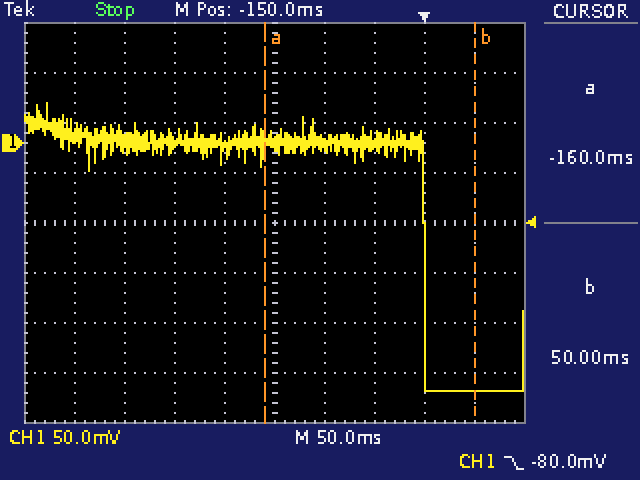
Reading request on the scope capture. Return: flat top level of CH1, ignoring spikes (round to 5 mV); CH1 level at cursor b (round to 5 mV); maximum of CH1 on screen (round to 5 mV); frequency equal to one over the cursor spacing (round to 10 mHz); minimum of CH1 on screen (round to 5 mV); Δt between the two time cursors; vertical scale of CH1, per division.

0 mV
-250 mV
40 mV
4.76 Hz
-250 mV
210 ms
50 mV
